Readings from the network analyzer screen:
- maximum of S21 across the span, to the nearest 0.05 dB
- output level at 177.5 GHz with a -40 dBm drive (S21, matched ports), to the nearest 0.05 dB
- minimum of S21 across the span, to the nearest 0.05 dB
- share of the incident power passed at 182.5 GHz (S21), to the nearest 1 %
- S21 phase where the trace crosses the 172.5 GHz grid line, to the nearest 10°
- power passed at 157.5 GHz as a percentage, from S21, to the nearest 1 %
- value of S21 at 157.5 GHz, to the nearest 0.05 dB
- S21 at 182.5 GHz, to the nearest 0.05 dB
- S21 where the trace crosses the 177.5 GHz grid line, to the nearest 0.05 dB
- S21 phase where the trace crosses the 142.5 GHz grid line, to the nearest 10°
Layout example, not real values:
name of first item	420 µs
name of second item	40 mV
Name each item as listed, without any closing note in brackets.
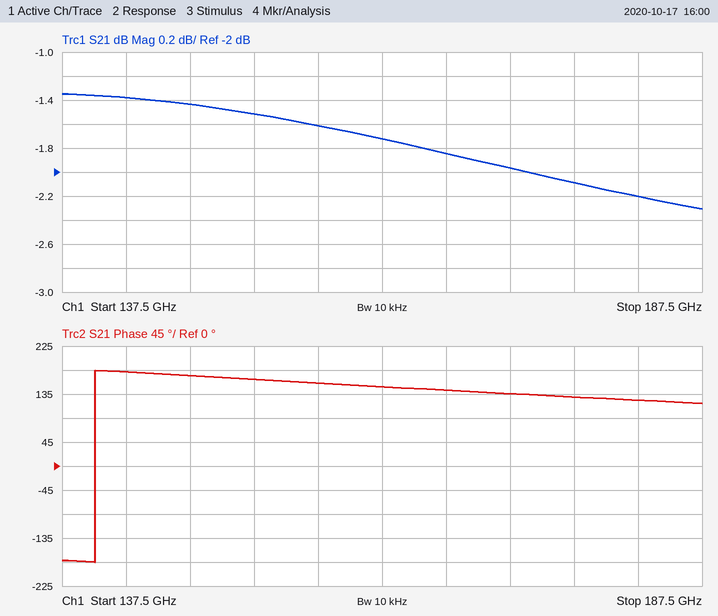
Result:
maximum of S21 across the span, to the nearest 0.05 dB	-1.35 dB
output level at 177.5 GHz with a -40 dBm drive (S21, matched ports), to the nearest 0.05 dB	-42.10 dBm
minimum of S21 across the span, to the nearest 0.05 dB	-2.30 dB
share of the incident power passed at 182.5 GHz (S21), to the nearest 1 %	60 %
S21 phase where the trace crosses the 172.5 GHz grid line, to the nearest 10°	140°
power passed at 157.5 GHz as a percentage, from S21, to the nearest 1 %	69 %
value of S21 at 157.5 GHz, to the nearest 0.05 dB	-1.60 dB
S21 at 182.5 GHz, to the nearest 0.05 dB	-2.20 dB
S21 where the trace crosses the 177.5 GHz grid line, to the nearest 0.05 dB	-2.10 dB
S21 phase where the trace crosses the 142.5 GHz grid line, to the nearest 10°	180°
